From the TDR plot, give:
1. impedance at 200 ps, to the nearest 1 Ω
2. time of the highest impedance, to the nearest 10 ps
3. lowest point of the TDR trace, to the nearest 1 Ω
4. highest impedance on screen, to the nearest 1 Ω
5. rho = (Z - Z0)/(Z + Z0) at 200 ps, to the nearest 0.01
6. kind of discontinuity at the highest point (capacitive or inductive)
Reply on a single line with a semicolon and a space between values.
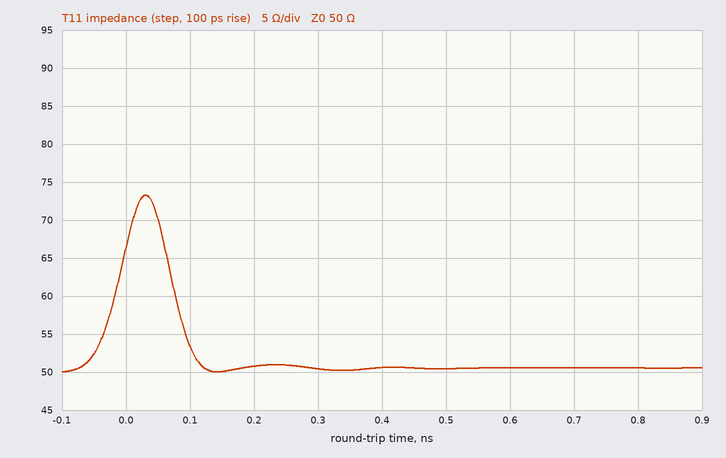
51 Ω; 30 ps; 50 Ω; 73 Ω; +0.01; inductive
